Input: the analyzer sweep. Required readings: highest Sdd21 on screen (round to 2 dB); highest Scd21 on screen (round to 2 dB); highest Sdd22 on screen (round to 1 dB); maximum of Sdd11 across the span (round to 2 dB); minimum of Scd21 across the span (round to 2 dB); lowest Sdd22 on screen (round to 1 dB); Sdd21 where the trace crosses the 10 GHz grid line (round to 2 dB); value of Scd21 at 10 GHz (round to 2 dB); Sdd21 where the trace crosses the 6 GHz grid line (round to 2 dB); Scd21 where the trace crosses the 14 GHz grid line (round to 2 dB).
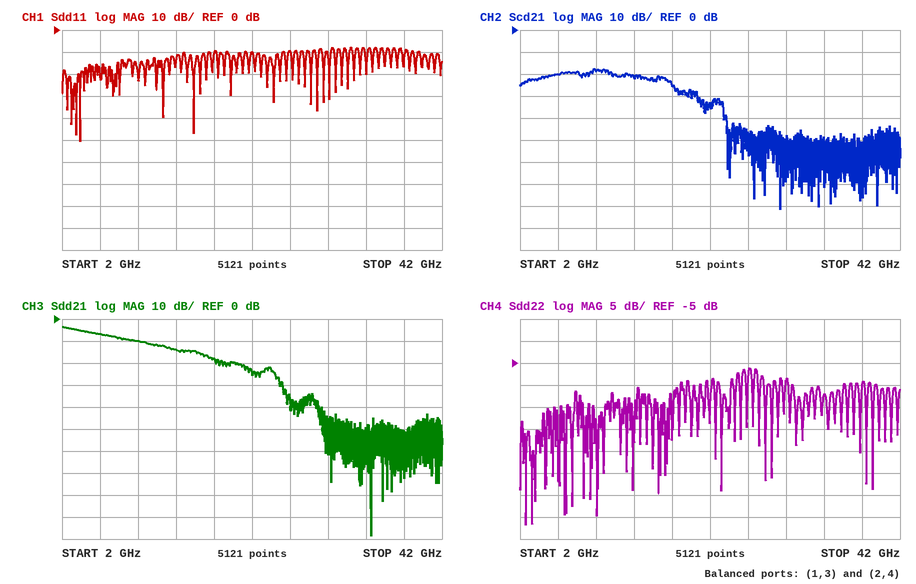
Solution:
-4 dB
-18 dB
-6 dB
-8 dB
-82 dB
-42 dB
-10 dB
-18 dB
-6 dB
-22 dB
